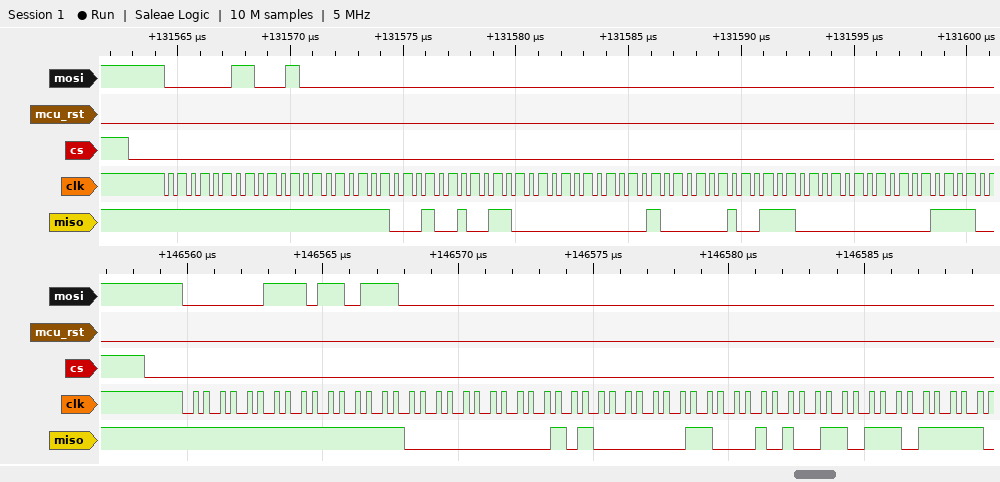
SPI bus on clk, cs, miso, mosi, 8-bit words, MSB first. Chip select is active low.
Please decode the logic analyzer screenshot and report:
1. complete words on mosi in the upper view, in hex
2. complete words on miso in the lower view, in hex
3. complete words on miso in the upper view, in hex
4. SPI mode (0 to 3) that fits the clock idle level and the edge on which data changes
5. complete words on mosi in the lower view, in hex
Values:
03, 10, 00, 00, 00, 00, 00, 00, 00
FF, FF, 00, 14, 06, 29, BB
FF, FF, F1, 26, 00, 10, 27, 00, 0F
3
03, B7, 00, 00, 00, 00, 00
